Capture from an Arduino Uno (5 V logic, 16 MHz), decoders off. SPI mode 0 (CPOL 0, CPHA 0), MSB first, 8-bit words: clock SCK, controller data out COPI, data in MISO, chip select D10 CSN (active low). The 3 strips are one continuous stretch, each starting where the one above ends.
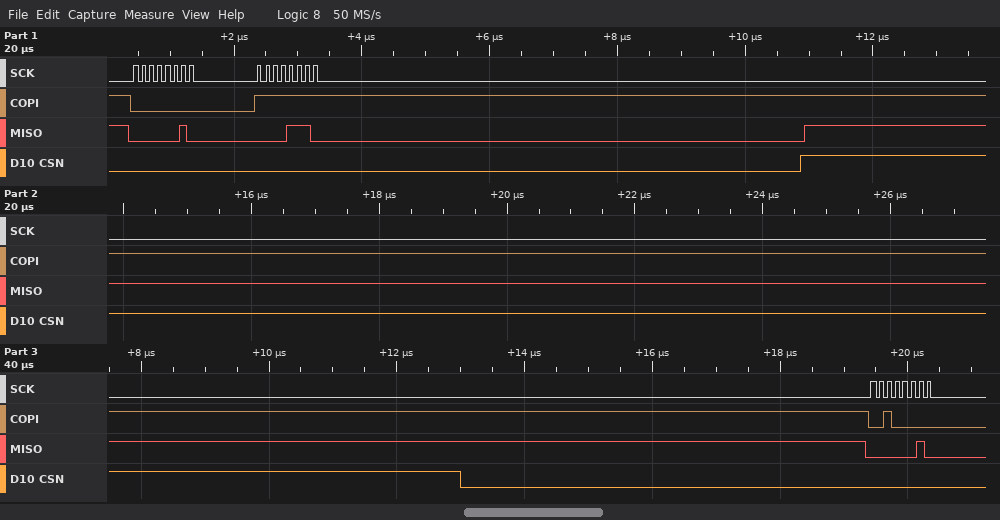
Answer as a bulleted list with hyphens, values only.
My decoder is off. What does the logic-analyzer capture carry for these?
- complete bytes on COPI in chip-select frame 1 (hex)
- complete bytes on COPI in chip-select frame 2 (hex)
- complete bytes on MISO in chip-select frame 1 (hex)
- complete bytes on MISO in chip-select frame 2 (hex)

- 00 FF
- 20
- 02 0E
- 02
